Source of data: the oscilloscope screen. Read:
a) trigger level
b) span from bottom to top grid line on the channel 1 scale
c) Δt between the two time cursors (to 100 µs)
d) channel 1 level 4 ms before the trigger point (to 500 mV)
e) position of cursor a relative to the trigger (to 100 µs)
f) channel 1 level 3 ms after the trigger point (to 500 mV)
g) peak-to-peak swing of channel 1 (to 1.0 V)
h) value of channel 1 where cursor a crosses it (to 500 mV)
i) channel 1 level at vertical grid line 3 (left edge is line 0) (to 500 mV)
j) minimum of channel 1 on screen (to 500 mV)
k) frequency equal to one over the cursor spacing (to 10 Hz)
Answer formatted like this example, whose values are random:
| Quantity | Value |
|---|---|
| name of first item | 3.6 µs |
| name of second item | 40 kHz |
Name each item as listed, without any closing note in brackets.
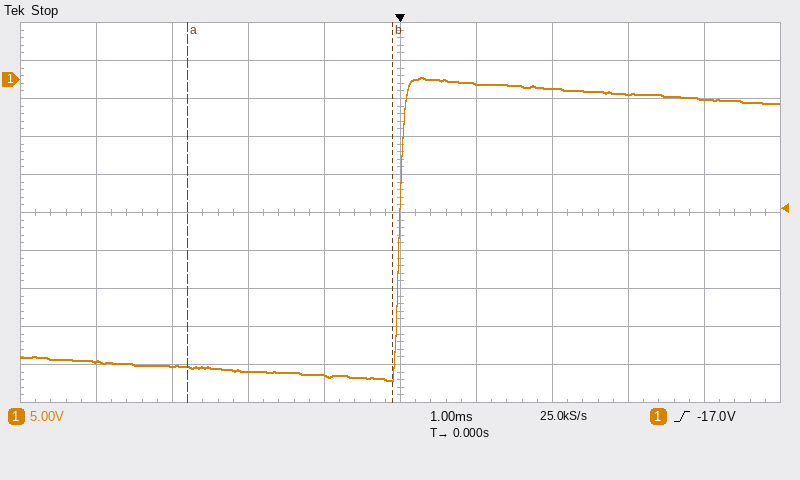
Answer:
| Quantity | Value |
|---|---|
| trigger level | -17.0 V |
| span from bottom to top grid line on the channel 1 scale | 50 V |
| Δt between the two time cursors | 2.7 ms |
| channel 1 level 4 ms before the trigger point | -37.0 V |
| position of cursor a relative to the trigger | -2.8 ms |
| channel 1 level 3 ms after the trigger point | -2.0 V |
| peak-to-peak swing of channel 1 | 40.0 V |
| value of channel 1 where cursor a crosses it | -38.0 V |
| channel 1 level at vertical grid line 3 (left edge is line 0) | -38.5 V |
| minimum of channel 1 on screen | -39.5 V |
| frequency equal to one over the cursor spacing | 370 Hz |
